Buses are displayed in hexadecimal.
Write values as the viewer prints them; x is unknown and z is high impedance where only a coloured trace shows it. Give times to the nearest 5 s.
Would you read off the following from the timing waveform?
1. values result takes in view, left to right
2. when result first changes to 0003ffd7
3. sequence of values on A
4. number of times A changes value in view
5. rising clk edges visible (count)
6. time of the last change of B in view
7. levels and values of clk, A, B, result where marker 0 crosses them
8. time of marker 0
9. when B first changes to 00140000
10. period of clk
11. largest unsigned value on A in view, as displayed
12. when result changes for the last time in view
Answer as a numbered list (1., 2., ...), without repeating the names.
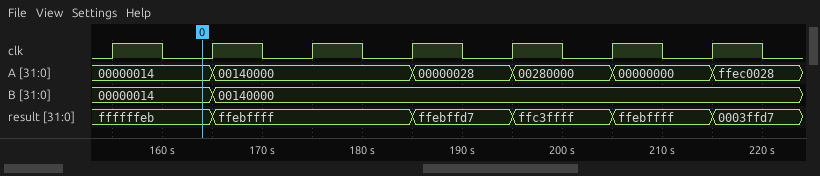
1. ffffffeb, ffebffff, ffebffd7, ffc3ffff, ffebffff, 0003ffd7
2. 215 s
3. 00000014, 00140000, 00000028, 00280000, 00000000, ffec0028
4. 5
5. 7
6. 165 s
7. clk=0, A=00000014, B=00000014, result=ffffffeb
8. 165 s
9. 165 s
10. 10 s
11. ffec0028
12. 215 s
